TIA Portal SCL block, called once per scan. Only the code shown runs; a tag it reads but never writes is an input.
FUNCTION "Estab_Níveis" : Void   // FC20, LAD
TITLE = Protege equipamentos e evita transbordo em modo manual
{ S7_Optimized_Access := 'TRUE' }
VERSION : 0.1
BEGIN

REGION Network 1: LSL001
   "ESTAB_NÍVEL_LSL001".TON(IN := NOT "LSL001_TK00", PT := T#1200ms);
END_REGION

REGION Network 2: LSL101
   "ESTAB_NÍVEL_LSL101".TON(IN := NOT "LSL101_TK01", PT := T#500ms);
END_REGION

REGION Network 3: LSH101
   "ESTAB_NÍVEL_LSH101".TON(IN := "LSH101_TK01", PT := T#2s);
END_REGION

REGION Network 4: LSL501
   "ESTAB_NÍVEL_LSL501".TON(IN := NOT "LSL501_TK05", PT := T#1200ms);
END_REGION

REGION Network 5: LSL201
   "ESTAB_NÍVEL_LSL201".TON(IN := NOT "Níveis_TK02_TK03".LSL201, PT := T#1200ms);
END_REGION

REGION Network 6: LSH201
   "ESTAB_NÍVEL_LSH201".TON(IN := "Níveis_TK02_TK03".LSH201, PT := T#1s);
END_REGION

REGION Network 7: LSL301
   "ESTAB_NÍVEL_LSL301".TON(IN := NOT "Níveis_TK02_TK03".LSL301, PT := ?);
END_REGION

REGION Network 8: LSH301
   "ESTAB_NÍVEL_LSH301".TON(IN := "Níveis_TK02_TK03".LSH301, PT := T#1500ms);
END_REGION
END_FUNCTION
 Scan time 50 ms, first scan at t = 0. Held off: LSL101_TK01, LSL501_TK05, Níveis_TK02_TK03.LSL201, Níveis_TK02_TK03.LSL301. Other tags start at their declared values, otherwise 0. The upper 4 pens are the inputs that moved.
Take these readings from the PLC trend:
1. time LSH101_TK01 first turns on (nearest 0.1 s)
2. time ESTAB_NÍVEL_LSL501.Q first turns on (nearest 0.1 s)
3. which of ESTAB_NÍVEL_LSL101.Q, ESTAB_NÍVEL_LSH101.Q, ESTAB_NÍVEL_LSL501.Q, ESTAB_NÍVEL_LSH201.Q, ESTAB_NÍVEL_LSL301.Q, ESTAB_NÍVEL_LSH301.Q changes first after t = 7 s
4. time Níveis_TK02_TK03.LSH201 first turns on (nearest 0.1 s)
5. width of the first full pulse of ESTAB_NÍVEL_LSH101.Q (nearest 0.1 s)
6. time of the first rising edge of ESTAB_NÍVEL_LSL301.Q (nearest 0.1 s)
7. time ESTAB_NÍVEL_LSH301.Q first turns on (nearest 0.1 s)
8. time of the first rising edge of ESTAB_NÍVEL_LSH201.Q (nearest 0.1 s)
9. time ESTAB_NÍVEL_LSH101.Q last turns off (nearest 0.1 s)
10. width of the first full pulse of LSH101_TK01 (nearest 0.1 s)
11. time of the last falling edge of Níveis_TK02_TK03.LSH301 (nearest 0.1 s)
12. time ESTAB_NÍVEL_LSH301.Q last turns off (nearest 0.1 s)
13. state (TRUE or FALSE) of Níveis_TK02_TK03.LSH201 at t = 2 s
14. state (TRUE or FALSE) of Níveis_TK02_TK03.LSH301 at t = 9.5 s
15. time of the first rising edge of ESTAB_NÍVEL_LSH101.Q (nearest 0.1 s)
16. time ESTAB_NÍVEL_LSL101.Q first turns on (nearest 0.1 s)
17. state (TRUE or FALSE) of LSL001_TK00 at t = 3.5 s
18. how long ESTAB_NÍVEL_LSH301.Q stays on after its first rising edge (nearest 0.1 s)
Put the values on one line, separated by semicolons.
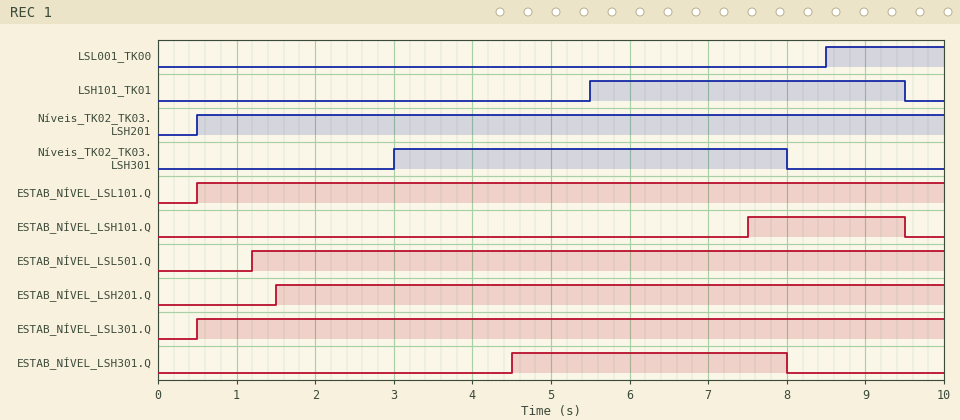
5.5 s; 1.2 s; ESTAB_NÍVEL_LSH101.Q; 0.5 s; 2.0 s; 0.5 s; 4.5 s; 1.5 s; 9.5 s; 4.0 s; 8.0 s; 8.0 s; TRUE; FALSE; 7.5 s; 0.5 s; FALSE; 3.5 s
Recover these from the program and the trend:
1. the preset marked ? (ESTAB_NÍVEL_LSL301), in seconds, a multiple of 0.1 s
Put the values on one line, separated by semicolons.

0.5 s
